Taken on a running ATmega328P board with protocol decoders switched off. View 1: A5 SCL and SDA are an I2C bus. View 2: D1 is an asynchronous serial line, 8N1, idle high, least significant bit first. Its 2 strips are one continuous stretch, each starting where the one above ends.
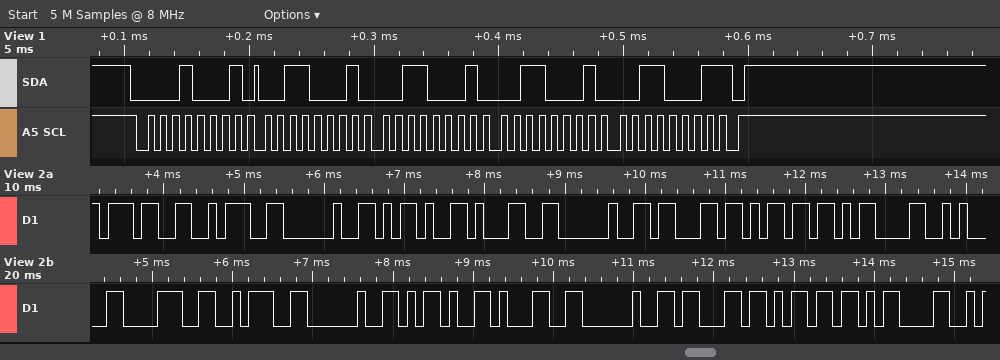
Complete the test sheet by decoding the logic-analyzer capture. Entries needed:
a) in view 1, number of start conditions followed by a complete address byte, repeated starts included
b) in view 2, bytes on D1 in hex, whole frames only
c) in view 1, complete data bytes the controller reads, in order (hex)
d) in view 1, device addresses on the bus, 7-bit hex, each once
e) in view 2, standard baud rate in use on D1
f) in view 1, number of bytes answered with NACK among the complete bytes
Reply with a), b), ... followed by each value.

a) 1
b) 37 3A 20 2D 31 20 63 6D 0D 0A 38 3A 20 2D 31 20 63 6D 0D
c) 31 31 31 31
d) 0x08
e) 9600 baud
f) 1
